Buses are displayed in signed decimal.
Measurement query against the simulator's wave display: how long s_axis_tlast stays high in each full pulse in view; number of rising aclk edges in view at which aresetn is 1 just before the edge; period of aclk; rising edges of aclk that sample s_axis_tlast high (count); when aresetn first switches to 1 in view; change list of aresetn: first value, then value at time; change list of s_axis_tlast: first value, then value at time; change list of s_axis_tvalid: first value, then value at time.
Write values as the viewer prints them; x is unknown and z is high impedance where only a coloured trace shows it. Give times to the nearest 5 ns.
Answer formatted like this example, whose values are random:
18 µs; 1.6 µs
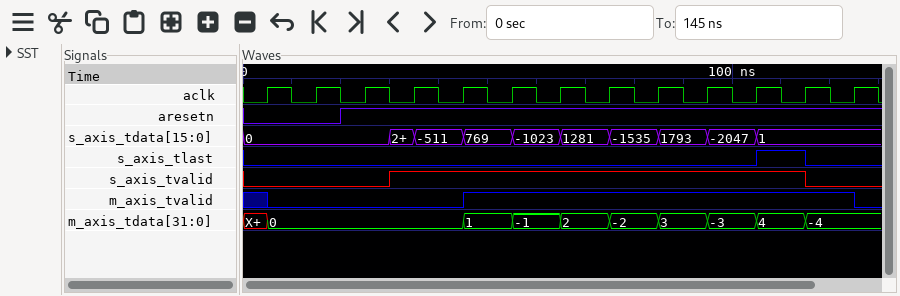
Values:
10 ns; 11; 10 ns; 1; 20 ns; 0, 1 at 20 ns; 0, 1 at 105 ns, 0 at 115 ns; 0, 1 at 30 ns, 0 at 115 ns
